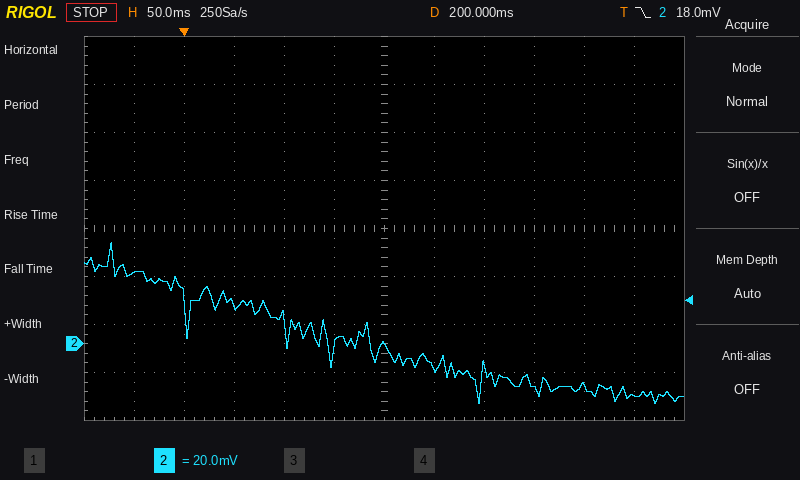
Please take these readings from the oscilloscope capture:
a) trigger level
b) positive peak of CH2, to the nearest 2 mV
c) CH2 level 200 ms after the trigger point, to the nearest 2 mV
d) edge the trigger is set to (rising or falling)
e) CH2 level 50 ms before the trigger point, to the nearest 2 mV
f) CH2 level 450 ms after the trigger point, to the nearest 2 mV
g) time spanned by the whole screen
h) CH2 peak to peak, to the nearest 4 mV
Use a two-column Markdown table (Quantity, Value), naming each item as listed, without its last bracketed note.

| Quantity | Value |
|---|---|
| trigger level | 18.0 mV |
| positive peak of CH2, to the nearest 2 mV | 42 mV |
| CH2 level 200 ms after the trigger point, to the nearest 2 mV | 0 mV |
| edge the trigger is set to | falling |
| CH2 level 50 ms before the trigger point, to the nearest 2 mV | 30 mV |
| CH2 level 450 ms after the trigger point, to the nearest 2 mV | -22 mV |
| time spanned by the whole screen | 600 ms |
| CH2 peak to peak, to the nearest 4 mV | 68 mV |
